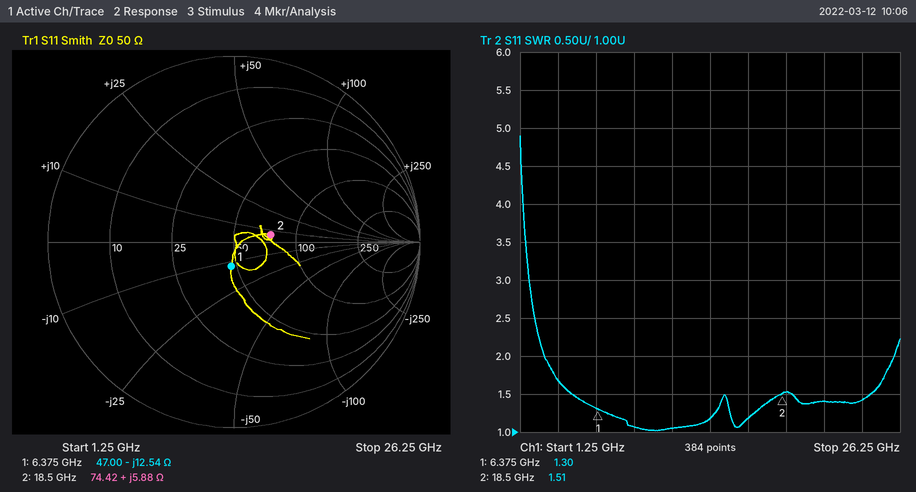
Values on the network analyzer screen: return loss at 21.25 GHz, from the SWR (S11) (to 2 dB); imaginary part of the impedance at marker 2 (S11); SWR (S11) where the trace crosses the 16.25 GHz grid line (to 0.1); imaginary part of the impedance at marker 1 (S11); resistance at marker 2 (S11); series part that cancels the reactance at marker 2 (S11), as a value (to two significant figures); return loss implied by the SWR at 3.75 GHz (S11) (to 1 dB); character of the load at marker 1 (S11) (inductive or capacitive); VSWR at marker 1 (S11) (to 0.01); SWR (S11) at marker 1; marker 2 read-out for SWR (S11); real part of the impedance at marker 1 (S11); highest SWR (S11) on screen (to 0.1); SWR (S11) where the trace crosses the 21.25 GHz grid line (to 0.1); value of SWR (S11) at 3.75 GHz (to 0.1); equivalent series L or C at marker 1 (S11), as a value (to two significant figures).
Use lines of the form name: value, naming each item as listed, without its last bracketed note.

return loss at 21.25 GHz, from the SWR (S11): 16 dB
imaginary part of the impedance at marker 2: +5.88 Ω
SWR (S11) where the trace crosses the 16.25 GHz grid line: 1.2
imaginary part of the impedance at marker 1: -12.54 Ω
resistance at marker 2: 74.42 Ω
series part that cancels the reactance at marker 2 (S11), as a value: 1.5 pF
return loss implied by the SWR at 3.75 GHz (S11): 12 dB
character of the load at marker 1 (S11): capacitive
VSWR at marker 1 (S11): 1.30
SWR (S11) at marker 1: 1.30
marker 2 read-out for SWR: 1.51
real part of the impedance at marker 1: 47.00 Ω
highest SWR (S11) on screen: 4.9
SWR (S11) where the trace crosses the 21.25 GHz grid line: 1.4
value of SWR (S11) at 3.75 GHz: 1.7
equivalent series L or C at marker 1 (S11), as a value: 2.0 pF
